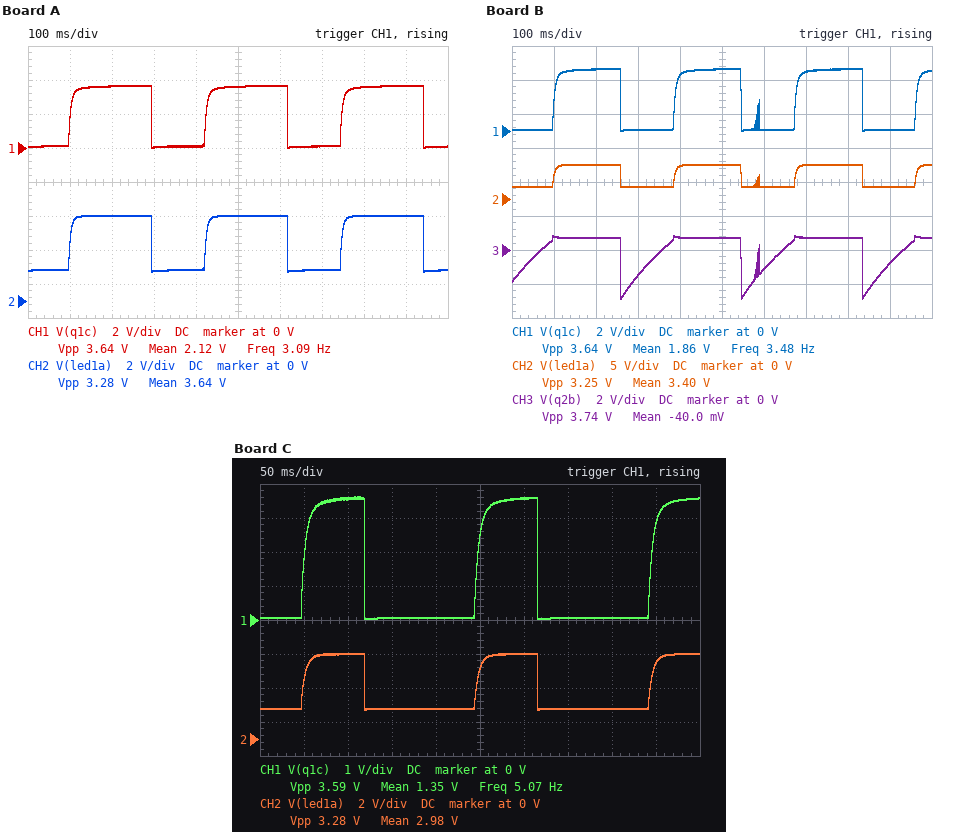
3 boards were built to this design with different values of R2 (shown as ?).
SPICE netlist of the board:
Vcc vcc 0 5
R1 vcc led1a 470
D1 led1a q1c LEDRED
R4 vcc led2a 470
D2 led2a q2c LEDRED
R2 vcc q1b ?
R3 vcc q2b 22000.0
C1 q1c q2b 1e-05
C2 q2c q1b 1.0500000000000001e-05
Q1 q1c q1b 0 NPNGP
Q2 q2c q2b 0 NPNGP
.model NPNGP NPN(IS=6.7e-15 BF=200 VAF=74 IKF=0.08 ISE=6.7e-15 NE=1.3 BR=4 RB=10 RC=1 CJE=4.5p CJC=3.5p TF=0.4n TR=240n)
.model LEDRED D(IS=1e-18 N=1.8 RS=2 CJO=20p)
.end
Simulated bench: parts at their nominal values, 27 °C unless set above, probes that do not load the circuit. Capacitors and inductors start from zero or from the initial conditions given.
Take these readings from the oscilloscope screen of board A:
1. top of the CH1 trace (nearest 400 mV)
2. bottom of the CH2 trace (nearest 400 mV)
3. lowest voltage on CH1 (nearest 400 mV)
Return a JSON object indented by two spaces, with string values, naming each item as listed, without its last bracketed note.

{
  "top of the CH1 trace": "3.6 V",
  "bottom of the CH2 trace": "1.6 V",
  "lowest voltage on CH1": "0 V"
}
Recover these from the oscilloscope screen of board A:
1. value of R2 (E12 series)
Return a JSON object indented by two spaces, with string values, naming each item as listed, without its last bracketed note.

{
  "value of R2": "33 kΩ"
}
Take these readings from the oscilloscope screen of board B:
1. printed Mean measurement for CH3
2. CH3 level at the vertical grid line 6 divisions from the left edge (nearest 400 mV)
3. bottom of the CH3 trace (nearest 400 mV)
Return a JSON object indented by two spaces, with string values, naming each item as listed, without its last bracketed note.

{
  "printed Mean measurement for CH3": "-40.0 mV",
  "CH3 level at the vertical grid line 6 divisions from the left edge": "-1.2 V",
  "bottom of the CH3 trace": "-2.8 V"
}
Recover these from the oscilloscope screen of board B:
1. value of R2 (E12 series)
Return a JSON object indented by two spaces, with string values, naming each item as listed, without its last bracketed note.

{
  "value of R2": "27 kΩ"
}
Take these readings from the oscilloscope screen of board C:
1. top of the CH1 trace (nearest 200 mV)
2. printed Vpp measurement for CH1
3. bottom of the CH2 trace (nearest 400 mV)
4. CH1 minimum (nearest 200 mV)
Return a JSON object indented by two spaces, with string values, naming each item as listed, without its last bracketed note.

{
  "top of the CH1 trace": "3.6 V",
  "printed Vpp measurement for CH1": "3.59 V",
  "bottom of the CH2 trace": "1.6 V",
  "CH1 minimum": "0 V"
}
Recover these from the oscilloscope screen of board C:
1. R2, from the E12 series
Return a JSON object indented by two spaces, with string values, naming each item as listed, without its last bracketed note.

{
  "R2, from the E12 series": "12 kΩ"
}
